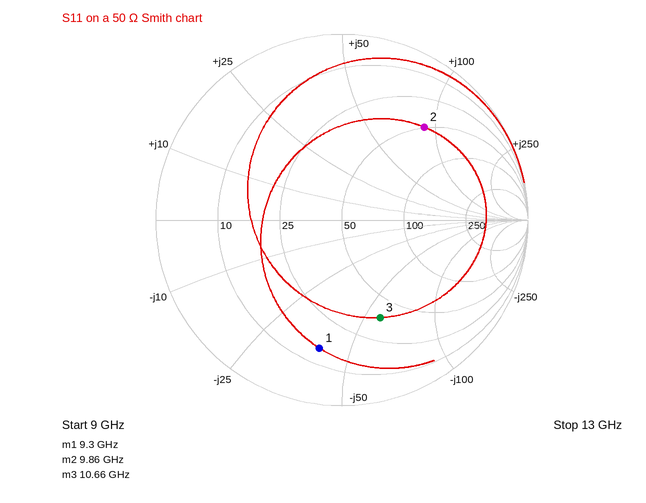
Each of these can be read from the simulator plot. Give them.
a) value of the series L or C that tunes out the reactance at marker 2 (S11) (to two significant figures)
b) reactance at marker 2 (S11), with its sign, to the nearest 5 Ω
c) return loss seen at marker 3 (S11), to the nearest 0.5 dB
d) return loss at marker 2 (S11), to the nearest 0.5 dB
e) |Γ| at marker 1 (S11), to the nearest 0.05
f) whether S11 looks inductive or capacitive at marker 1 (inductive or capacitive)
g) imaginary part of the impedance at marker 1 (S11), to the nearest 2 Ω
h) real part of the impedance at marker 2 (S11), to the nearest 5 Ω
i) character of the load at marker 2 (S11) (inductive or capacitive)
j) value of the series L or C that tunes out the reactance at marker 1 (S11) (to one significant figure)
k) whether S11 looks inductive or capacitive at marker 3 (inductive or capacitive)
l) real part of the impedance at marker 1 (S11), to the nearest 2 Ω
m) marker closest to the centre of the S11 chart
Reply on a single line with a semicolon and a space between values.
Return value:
180 fF; +90 Ω; 5.0 dB; 3.5 dB; 0.70; capacitive; -40 Ω; 50 Ω; inductive; 700 pH; capacitive; 14 Ω; marker 3
